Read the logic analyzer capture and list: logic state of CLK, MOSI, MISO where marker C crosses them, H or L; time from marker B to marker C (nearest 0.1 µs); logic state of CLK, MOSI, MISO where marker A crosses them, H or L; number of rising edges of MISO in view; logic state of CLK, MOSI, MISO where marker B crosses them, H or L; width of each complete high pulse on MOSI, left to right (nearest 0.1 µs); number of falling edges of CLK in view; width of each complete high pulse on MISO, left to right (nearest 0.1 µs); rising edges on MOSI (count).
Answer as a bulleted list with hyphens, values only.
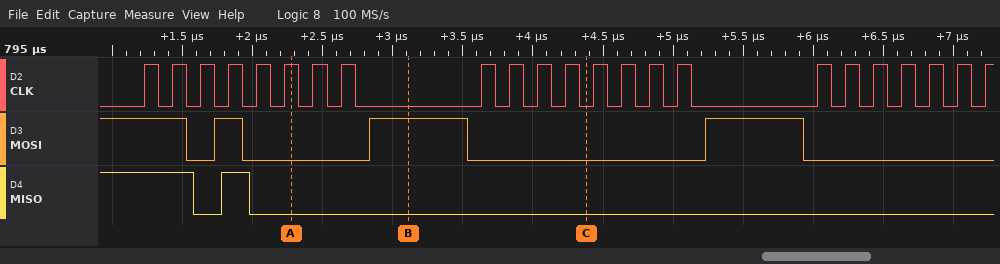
- CLK=L, MOSI=L, MISO=L
- 1.3 µs
- CLK=H, MOSI=L, MISO=L
- 1
- CLK=L, MOSI=H, MISO=L
- 0.2 µs, 0.7 µs, 0.7 µs
- 22
- 0.2 µs
- 3
